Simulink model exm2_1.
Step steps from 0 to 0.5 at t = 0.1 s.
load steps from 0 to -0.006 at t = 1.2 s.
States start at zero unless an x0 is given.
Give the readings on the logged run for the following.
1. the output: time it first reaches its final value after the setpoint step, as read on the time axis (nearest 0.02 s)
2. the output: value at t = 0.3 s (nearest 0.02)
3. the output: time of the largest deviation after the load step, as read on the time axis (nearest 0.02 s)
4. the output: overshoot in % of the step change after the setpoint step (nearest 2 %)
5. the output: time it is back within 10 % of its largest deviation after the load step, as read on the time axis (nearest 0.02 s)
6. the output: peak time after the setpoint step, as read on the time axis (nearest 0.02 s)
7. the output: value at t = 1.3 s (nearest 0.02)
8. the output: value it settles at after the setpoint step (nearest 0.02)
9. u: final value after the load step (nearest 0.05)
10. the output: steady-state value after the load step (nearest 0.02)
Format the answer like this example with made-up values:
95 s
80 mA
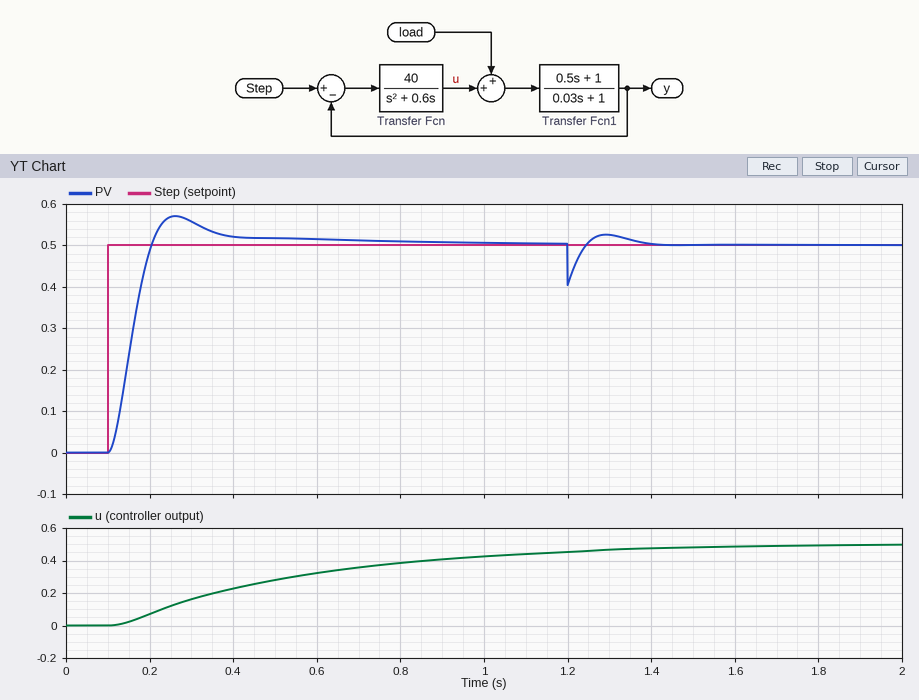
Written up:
0.20 s
0.56
1.20 s
14 %
1.36 s
0.26 s
0.52
0.50
0.50
0.50
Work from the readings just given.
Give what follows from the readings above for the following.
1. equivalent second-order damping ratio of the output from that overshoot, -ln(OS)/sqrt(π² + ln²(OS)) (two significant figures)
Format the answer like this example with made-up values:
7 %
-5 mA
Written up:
0.53
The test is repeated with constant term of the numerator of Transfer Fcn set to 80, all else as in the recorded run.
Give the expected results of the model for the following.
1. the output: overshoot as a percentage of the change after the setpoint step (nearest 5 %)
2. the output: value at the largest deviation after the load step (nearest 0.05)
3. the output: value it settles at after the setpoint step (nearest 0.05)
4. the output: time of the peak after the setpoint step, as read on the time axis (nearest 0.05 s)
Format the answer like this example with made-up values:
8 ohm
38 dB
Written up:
25 %
0.40
0.50
0.20 s
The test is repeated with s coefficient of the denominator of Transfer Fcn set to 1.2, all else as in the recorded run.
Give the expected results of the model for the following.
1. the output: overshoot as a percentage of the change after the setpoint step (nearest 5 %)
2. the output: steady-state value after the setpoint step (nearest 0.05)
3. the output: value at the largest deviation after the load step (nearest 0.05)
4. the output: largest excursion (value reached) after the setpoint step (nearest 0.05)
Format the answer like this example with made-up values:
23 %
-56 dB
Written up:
10 %
0.50
0.40
0.55
